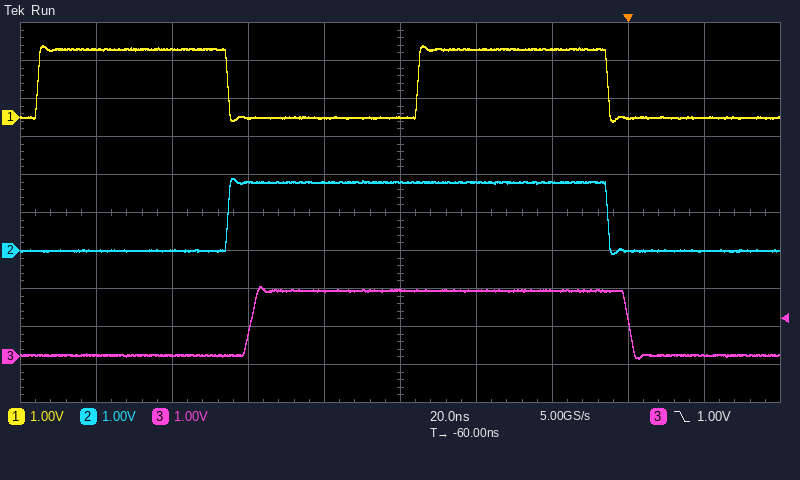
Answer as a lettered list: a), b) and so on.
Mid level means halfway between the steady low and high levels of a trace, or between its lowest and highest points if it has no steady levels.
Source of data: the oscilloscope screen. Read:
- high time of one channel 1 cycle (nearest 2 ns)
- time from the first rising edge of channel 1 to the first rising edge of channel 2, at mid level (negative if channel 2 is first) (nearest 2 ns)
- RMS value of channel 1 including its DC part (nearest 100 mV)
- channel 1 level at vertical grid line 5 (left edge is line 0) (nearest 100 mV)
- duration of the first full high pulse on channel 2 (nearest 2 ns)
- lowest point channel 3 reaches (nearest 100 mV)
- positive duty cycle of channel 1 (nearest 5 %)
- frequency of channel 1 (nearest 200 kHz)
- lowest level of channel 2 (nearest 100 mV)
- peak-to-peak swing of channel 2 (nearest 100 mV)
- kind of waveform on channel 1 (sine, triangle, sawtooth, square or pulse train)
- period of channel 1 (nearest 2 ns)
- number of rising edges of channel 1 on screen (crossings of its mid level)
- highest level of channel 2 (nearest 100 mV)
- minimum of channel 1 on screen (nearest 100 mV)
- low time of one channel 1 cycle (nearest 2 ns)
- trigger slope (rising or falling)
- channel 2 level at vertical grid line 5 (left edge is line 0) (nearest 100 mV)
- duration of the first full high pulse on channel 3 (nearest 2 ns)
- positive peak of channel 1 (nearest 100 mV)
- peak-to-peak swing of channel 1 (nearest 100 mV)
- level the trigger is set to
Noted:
a) 50 ns
b) +50 ns
c) 1.3 V
d) 0.0 V
e) 100 ns
f) 0.0 V
g) 50 %
h) 10.0 MHz
i) -100 mV
j) 2.0 V
k) square
l) 100 ns
m) 2
n) 1.9 V
o) -100 mV
p) 50 ns
q) falling
r) 1.8 V
s) 100 ns
t) 1.9 V
u) 2.0 V
v) 1.00 V
